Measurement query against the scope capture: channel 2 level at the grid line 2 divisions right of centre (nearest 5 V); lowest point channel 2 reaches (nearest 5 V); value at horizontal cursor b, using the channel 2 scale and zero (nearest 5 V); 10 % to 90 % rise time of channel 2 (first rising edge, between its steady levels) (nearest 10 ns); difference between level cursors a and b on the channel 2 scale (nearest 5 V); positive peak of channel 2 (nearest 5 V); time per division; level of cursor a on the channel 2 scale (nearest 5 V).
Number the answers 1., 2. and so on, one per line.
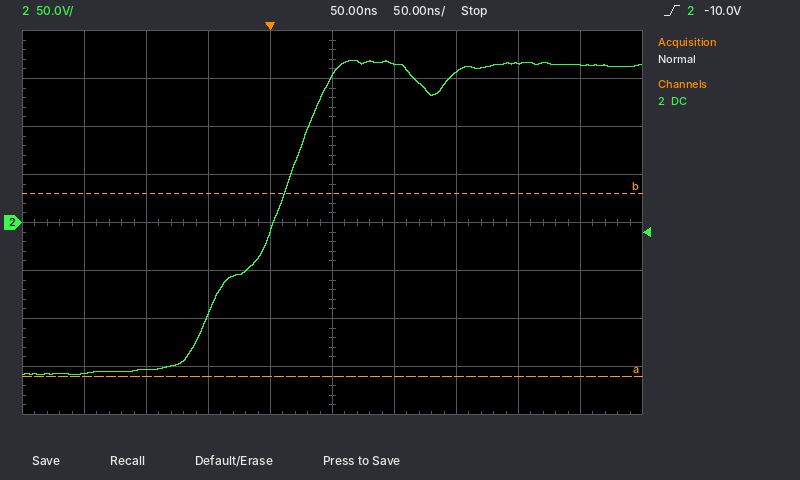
1. 155 V
2. -160 V
3. 30 V
4. 100 ns
5. 190 V
6. 170 V
7. 50 ns
8. -160 V
